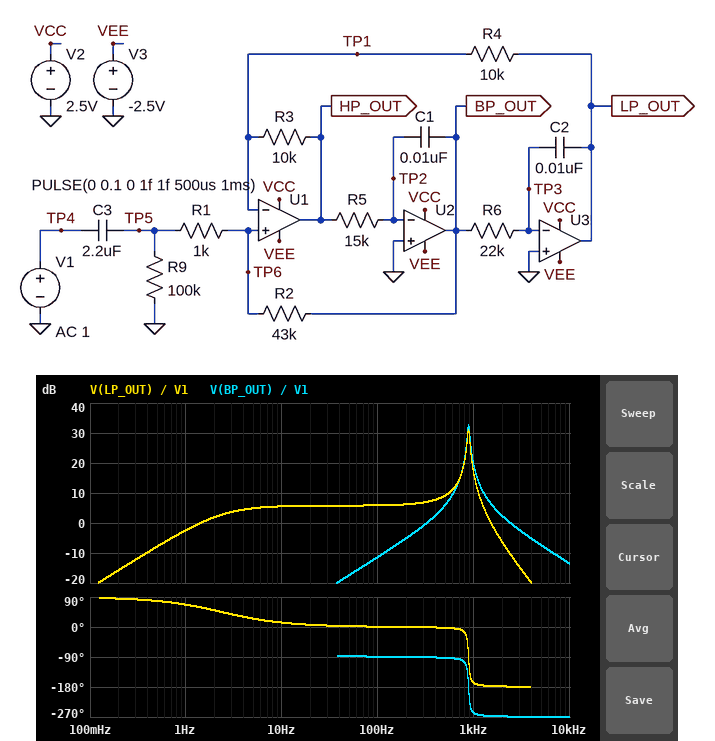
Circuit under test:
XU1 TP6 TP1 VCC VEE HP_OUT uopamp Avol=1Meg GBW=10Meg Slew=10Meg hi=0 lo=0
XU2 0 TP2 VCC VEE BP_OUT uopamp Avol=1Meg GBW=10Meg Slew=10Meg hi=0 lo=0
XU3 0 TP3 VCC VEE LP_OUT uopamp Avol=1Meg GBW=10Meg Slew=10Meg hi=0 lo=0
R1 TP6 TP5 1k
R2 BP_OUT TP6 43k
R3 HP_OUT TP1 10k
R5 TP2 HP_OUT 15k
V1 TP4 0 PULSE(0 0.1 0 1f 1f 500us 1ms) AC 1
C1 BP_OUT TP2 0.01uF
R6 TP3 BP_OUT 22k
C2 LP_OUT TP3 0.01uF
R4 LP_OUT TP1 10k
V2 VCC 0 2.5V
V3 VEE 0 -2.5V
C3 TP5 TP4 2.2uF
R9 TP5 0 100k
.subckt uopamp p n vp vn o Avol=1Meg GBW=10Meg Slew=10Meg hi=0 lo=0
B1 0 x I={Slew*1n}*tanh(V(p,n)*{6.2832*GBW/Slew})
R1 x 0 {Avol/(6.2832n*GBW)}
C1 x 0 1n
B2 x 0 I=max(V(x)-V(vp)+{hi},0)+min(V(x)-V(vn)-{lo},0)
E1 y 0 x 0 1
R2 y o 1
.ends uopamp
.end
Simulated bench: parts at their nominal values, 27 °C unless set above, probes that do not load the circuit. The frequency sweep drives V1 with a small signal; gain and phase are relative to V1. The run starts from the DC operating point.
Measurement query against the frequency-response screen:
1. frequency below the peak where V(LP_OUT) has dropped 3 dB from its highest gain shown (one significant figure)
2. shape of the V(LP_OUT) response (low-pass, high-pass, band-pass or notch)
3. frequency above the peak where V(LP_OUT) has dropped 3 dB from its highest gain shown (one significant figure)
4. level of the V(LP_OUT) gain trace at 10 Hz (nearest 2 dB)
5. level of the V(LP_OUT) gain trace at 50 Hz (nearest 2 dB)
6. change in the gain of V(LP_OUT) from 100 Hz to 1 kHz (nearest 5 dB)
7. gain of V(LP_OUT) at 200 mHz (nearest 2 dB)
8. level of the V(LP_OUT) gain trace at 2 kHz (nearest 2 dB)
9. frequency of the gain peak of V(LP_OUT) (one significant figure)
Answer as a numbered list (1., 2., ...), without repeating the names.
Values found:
1. 900 Hz
2. band-pass
3. 900 Hz
4. 6 dB
5. 6 dB
6. 10 dB
7. -16 dB
8. -6 dB
9. 900 Hz
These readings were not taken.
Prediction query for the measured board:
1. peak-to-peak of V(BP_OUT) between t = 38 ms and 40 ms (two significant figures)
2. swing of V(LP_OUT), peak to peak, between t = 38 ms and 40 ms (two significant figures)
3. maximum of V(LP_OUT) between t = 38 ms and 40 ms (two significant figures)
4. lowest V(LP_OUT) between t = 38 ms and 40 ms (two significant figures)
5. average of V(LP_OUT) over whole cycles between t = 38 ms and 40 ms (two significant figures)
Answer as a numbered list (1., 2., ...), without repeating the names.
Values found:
1. 1.2 V
2. 810 mV
3. 460 mV
4. -350 mV
5. 55 mV
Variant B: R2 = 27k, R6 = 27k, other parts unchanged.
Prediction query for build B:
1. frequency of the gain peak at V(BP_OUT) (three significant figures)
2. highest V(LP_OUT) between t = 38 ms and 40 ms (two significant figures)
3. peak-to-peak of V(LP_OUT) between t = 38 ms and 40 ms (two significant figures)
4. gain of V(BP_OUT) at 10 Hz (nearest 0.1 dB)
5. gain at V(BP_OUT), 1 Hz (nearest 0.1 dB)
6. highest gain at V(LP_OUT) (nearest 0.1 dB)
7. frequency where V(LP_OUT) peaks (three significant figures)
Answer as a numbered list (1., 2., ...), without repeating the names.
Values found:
1. 794 Hz
2. 240 mV
3. 400 mV
4. -30.2 dB
5. -60.5 dB
6. 26.1 dB
7. 792 Hz
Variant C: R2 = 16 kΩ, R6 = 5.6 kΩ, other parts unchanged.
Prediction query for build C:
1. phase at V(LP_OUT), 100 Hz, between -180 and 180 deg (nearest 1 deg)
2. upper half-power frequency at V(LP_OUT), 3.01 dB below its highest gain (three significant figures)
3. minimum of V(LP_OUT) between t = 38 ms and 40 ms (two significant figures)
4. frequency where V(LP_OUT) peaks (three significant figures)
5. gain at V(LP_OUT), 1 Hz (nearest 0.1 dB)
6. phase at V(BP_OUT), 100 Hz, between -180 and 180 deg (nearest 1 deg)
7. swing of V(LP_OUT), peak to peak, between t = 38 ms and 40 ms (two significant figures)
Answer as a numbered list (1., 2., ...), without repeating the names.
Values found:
1. 3 deg
2. 1.80 kHz
3. -170 mV
4. 1.74 kHz
5. -8.6 dB
6. -87 deg
7. 390 mV
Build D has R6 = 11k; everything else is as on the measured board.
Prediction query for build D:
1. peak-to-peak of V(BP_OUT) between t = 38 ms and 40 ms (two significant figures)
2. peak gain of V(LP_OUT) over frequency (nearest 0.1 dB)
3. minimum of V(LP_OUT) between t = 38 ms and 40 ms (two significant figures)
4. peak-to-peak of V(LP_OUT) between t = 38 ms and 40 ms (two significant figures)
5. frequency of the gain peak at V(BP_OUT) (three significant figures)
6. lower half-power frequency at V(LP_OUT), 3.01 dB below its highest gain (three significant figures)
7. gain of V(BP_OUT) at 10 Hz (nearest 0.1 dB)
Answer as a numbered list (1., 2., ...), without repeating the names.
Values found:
1. 470 mV
2. 34.1 dB
3. -310 mV
4. 720 mV
5. 1.24 kHz
6. 1.22 kHz
7. -37.6 dB
